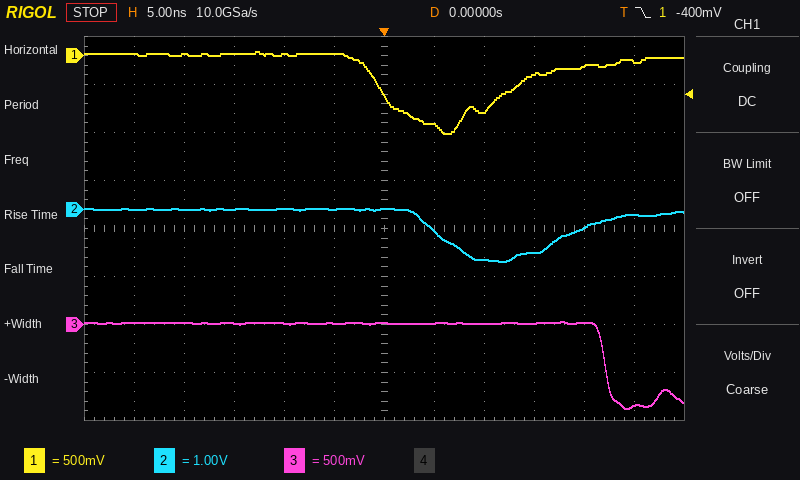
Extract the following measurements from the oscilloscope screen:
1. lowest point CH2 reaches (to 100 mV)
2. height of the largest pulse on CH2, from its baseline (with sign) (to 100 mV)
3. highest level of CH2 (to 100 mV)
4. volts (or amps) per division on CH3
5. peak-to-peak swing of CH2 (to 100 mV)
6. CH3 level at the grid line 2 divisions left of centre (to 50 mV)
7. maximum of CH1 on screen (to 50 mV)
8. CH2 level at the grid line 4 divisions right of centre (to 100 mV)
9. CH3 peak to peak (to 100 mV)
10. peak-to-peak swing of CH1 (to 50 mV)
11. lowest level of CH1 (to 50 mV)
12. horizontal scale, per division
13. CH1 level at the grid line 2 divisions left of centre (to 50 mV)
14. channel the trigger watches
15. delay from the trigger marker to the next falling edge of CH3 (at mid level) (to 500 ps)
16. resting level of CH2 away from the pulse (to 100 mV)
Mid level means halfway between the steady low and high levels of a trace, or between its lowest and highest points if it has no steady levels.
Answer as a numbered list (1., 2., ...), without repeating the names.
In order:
1. -1.1 V
2. -1.1 V
3. 0.0 V
4. 500 mV
5. 1.1 V
6. 0 mV
7. 50 mV
8. -400 mV
9. 900 mV
10. 850 mV
11. -800 mV
12. 5 ns
13. 0 mV
14. CH1
15. 22.0 ns
16. 0.0 V
